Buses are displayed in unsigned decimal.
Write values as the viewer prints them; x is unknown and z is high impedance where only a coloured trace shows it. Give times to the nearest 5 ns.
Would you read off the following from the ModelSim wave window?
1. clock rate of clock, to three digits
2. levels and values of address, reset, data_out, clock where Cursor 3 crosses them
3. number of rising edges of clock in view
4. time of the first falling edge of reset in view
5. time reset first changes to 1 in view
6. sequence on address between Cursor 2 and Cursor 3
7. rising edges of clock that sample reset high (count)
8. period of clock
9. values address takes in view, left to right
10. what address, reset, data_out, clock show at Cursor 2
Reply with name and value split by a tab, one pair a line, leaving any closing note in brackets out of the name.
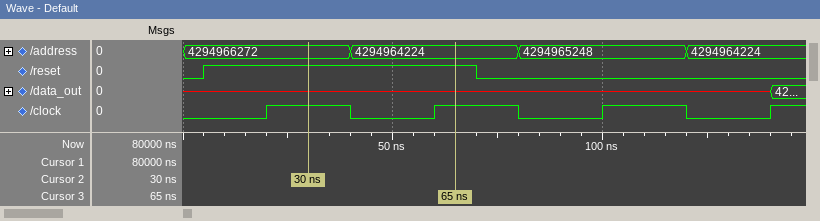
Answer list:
clock rate of clock, to three digits	25.0 MHz
levels and values of address, reset, data_out, clock where Cursor 3 crosses them	address=4294964224, reset=1, data_out=x, clock=1
number of rising edges of clock in view	4
time of the first falling edge of reset in view	70 ns
time reset first changes to 1 in view	5 ns
sequence on address between Cursor 2 and Cursor 3	4294966272, 4294964224
rising edges of clock that sample reset high	2
period of clock	40 ns
values address takes in view, left to right	4294966272, 4294964224, 4294965248, 4294964224
what address, reset, data_out, clock show at Cursor 2	address=4294966272, reset=1, data_out=x, clock=1
